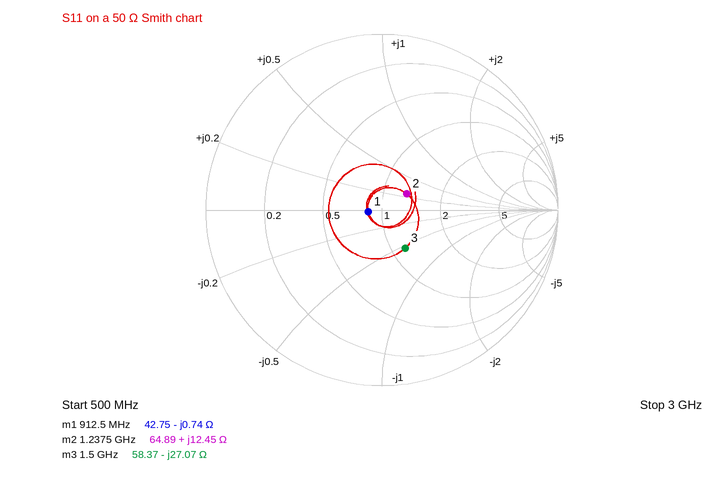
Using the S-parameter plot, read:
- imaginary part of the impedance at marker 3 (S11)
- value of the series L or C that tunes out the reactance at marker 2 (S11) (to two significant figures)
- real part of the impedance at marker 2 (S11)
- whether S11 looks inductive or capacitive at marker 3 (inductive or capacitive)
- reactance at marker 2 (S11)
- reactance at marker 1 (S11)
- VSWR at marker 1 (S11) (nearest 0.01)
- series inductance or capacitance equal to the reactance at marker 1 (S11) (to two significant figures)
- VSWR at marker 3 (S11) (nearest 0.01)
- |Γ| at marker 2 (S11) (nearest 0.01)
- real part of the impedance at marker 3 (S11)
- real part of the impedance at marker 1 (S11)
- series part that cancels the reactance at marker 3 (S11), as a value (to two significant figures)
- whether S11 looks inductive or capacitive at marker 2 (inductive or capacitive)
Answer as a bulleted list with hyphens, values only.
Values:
- -27.07 Ω
- 10 pF
- 64.89 Ω
- capacitive
- +12.45 Ω
- -0.74 Ω
- 1.17
- 240 pF
- 1.68
- 0.17
- 58.37 Ω
- 42.75 Ω
- 2.9 nH
- inductive
